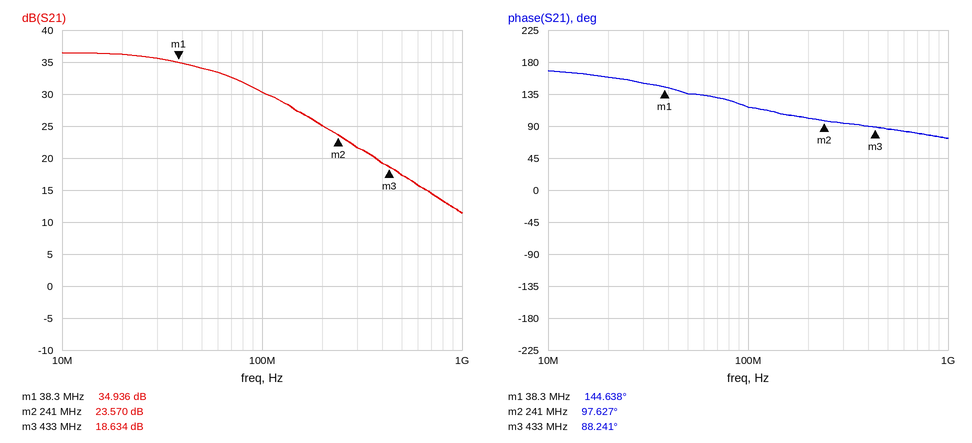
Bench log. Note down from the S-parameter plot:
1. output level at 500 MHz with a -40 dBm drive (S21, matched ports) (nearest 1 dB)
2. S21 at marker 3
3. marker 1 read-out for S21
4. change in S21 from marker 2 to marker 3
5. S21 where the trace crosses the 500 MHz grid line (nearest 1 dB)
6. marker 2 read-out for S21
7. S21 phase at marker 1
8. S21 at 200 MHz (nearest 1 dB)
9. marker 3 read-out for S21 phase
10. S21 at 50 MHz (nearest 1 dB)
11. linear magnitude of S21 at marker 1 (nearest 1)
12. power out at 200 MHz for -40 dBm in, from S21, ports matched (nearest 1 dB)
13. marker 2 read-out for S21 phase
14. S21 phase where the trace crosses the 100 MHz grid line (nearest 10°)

-23 dBm
18.634 dB
34.936 dB
-4.936 dB
17 dB
23.570 dB
144.638°
25 dB
88.241°
34 dB
56
-15 dBm
97.627°
120°
